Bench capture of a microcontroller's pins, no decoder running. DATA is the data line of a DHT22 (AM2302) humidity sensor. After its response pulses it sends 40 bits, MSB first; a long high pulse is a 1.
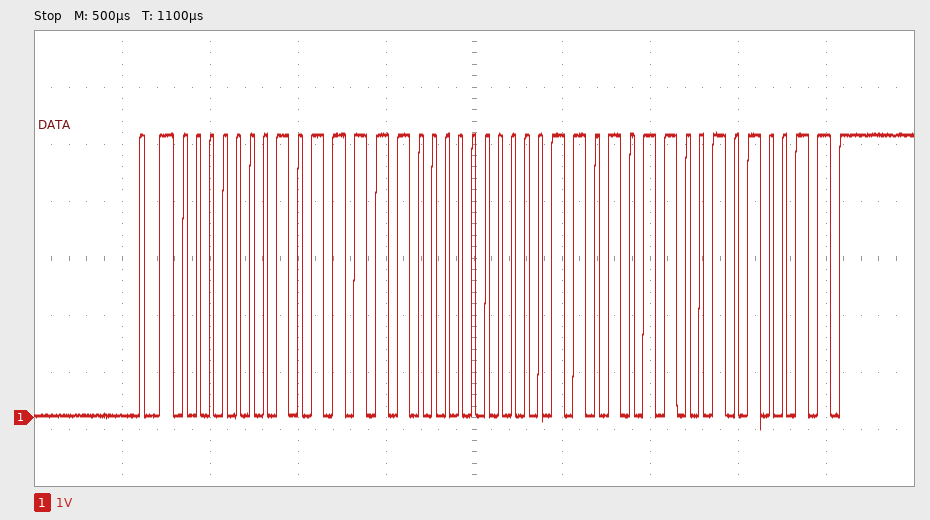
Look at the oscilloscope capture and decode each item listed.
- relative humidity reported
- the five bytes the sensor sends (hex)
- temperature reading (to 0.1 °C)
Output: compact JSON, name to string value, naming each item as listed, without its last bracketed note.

{"relative humidity reported": "38.0 %", "the five bytes the sensor sends": "01 7C 00 D6 53", "temperature reading": "21.4 °C"}
